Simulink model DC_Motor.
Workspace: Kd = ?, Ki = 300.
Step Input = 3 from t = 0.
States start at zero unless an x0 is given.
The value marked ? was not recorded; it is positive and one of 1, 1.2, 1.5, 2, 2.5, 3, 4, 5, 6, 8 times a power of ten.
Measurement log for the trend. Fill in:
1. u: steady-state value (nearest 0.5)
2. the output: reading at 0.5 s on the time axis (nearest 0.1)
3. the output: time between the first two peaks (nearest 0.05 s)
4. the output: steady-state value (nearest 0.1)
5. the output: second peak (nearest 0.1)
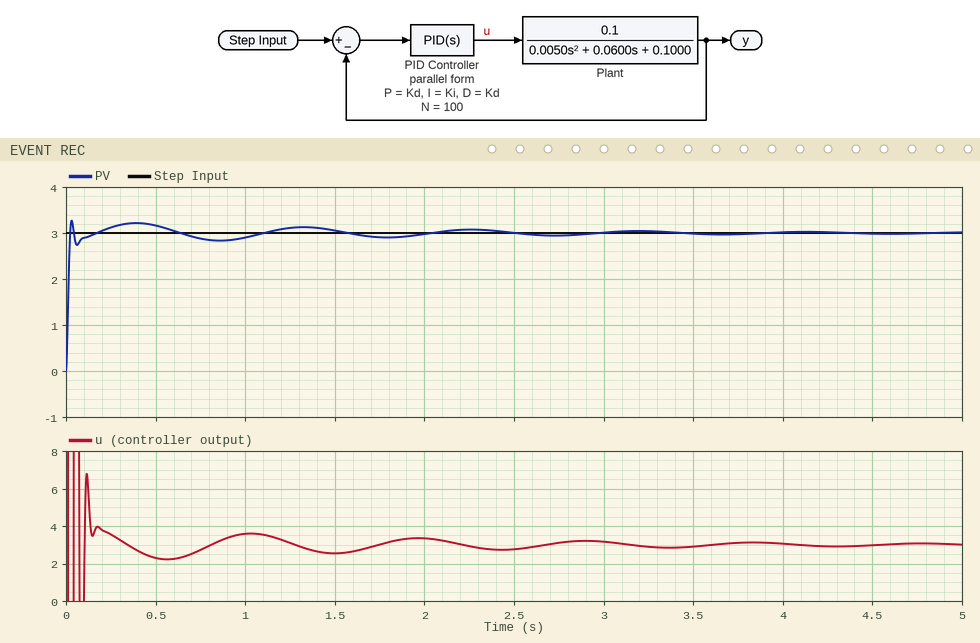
3.0
3.2
0.35 s
3.0
3.2
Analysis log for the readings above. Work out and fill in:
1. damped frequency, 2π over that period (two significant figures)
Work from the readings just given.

18 rad/s
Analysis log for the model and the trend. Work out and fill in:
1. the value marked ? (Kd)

6
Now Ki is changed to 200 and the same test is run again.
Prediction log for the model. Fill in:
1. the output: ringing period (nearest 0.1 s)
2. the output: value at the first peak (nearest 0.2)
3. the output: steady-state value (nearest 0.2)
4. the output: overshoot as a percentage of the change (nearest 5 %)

0.5 s
3.2
3.0
10 %
